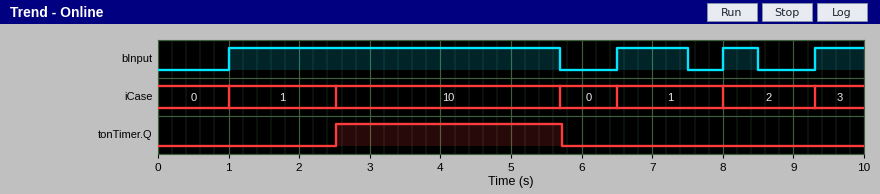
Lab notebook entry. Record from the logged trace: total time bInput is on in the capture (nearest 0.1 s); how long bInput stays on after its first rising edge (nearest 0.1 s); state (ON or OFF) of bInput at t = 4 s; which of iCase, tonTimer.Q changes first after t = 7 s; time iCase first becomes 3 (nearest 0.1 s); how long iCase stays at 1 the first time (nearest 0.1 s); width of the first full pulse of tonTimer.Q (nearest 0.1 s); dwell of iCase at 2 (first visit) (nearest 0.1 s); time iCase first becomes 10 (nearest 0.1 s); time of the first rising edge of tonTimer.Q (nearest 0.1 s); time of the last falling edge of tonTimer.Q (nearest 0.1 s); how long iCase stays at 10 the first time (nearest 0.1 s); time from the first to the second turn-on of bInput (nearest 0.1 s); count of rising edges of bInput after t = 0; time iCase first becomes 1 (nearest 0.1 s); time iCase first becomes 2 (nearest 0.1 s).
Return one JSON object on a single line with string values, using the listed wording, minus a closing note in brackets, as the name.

{"total time bInput is on in the capture": "6.9 s", "how long bInput stays on after its first rising edge": "4.7 s", "state (ON or OFF) of bInput at t = 4 s": "ON", "which of iCase, tonTimer.Q changes first after t = 7 s": "iCase", "time iCase first becomes 3": "9.3 s", "how long iCase stays at 1 the first time": "1.5 s", "width of the first full pulse of tonTimer.Q": "3.2 s", "dwell of iCase at 2 (first visit)": "1.3 s", "time iCase first becomes 10": "2.5 s", "time of the first rising edge of tonTimer.Q": "2.5 s", "time of the last falling edge of tonTimer.Q": "5.7 s", "how long iCase stays at 10 the first time": "3.2 s", "time from the first to the second turn-on of bInput": "5.5 s", "count of rising edges of bInput after t = 0": "4", "time iCase first becomes 1": "1.0 s", "time iCase first becomes 2": "8.0 s"}
